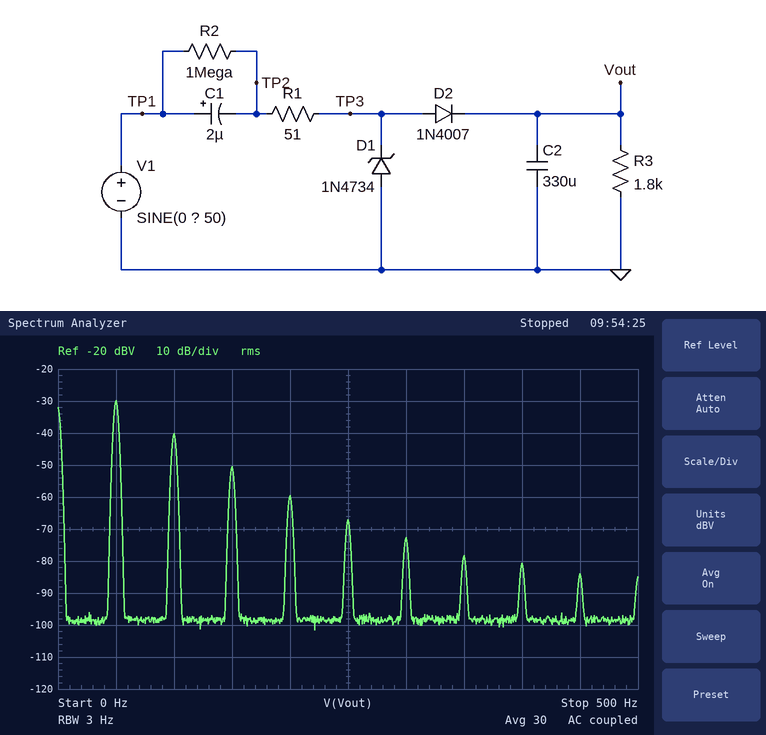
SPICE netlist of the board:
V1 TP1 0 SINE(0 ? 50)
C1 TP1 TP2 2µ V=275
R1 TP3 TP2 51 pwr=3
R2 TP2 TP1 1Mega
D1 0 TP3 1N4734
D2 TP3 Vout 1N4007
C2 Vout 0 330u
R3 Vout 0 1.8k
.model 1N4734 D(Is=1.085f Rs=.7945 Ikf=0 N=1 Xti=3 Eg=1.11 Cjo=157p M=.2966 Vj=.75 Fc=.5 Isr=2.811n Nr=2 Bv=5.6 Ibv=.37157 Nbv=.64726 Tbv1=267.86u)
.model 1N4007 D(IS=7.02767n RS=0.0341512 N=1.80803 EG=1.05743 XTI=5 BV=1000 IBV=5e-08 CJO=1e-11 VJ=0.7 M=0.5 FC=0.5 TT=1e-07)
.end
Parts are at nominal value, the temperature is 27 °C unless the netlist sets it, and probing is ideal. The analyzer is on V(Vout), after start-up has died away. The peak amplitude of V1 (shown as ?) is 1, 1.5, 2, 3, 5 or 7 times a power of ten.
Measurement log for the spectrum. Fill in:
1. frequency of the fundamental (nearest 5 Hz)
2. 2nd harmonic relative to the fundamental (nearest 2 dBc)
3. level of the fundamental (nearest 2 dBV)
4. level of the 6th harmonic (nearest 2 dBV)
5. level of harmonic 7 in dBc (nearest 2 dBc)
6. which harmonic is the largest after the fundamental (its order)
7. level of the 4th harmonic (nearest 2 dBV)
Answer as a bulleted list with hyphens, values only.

- 50 Hz
- -10 dBc
- -30 dBV
- -72 dBV
- -48 dBc
- 2
- -60 dBV
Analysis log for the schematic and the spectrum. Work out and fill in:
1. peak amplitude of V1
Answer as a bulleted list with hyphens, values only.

- 300 V
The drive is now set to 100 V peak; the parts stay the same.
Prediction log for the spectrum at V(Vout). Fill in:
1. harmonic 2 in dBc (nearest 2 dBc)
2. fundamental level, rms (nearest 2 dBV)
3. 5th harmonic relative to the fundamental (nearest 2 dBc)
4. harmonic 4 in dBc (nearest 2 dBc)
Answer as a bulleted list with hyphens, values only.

- -12 dBc
- -30 dBV
- -30 dBc
- -24 dBc
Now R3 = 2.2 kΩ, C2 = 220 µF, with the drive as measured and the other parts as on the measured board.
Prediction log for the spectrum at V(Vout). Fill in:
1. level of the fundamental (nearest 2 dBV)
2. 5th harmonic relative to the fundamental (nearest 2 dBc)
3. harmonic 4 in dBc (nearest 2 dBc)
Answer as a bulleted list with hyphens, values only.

- -28 dBV
- -34 dBc
- -28 dBc
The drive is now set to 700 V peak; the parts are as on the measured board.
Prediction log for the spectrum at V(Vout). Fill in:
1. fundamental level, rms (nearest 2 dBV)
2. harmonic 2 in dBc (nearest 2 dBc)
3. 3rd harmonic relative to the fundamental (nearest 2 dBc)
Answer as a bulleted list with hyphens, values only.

- -28 dBV
- -8 dBc
- -16 dBc
